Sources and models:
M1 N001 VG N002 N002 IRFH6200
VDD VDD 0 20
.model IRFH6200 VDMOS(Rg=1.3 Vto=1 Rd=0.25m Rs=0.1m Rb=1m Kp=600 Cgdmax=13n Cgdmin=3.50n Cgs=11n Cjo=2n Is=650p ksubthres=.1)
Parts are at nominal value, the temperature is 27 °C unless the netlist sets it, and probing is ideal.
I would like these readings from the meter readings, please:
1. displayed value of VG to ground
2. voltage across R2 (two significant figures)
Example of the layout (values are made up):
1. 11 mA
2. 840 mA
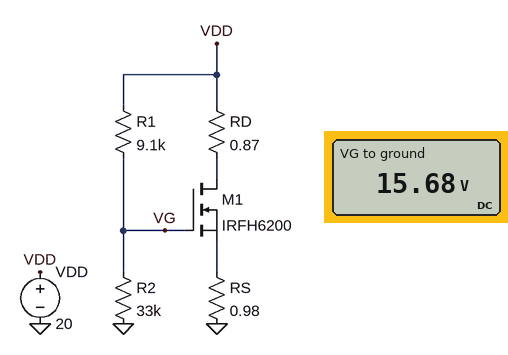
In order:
1. 15.68 V
2. 16 V
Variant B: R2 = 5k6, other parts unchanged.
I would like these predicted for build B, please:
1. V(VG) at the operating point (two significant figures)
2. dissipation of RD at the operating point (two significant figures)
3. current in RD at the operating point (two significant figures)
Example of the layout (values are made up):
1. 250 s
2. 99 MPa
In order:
1. 7.6 V
2. 38 W
3. 6.6 A
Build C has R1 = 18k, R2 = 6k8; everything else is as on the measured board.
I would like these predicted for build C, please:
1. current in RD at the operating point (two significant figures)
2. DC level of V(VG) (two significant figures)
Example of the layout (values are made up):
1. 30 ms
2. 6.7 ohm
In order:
1. 4.5 A
2. 5.5 V
